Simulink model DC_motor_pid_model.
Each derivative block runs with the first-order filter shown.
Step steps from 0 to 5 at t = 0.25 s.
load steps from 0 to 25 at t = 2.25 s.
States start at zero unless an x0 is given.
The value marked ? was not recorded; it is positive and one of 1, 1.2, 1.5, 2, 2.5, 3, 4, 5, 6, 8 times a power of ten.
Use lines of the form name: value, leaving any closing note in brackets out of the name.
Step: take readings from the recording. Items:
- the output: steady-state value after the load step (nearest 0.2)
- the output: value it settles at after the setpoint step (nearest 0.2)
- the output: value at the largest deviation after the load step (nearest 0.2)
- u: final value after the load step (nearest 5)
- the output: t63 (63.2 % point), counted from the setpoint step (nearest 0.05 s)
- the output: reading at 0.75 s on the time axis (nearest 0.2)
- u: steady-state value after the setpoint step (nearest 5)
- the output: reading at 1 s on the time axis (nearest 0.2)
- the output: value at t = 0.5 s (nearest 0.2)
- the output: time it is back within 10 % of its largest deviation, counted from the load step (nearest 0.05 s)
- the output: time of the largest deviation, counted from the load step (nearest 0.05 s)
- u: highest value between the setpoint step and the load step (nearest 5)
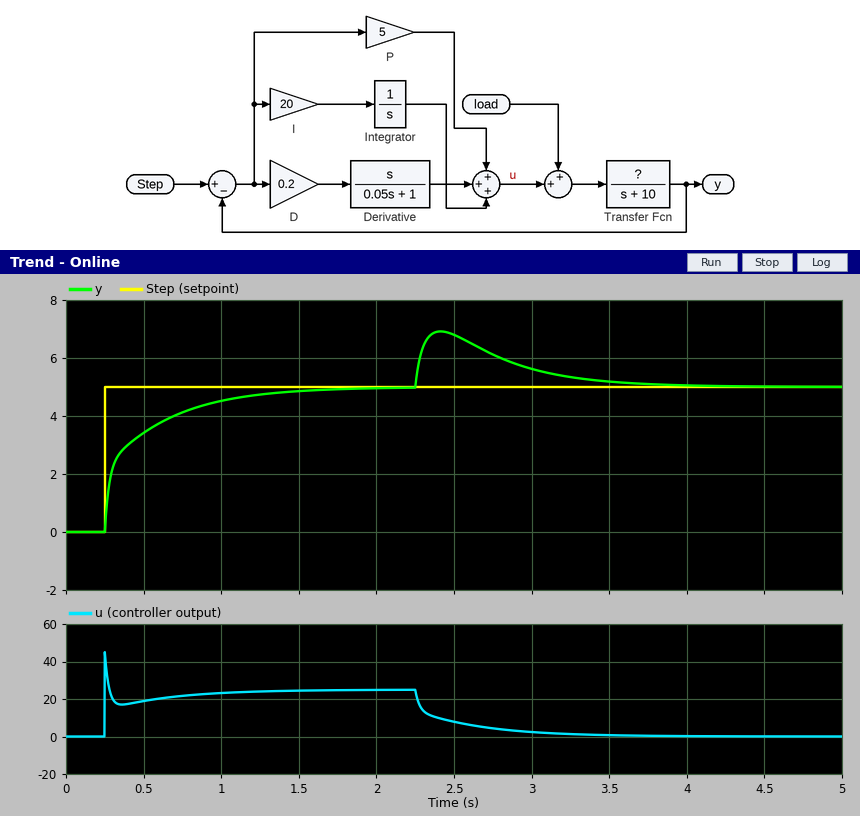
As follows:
the output: steady-state value after the load step: 5.0
the output: value it settles at after the setpoint step: 5.0
the output: value at the largest deviation after the load step: 7.0
u: final value after the load step: 0
the output: t63 (63.2 % point), counted from the setpoint step: 0.20 s
the output: reading at 0.75 s on the time axis: 4.2
u: steady-state value after the setpoint step: 25
the output: reading at 1 s on the time axis: 4.6
the output: value at t = 0.5 s: 3.4
the output: time it is back within 10 % of its largest deviation, counted from the load step: 1.25 s
the output: time of the largest deviation, counted from the load step: 0.15 s
u: highest value between the setpoint step and the load step: 45
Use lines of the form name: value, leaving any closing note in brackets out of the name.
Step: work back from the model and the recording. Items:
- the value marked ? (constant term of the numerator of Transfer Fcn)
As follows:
the value marked ?: 2
